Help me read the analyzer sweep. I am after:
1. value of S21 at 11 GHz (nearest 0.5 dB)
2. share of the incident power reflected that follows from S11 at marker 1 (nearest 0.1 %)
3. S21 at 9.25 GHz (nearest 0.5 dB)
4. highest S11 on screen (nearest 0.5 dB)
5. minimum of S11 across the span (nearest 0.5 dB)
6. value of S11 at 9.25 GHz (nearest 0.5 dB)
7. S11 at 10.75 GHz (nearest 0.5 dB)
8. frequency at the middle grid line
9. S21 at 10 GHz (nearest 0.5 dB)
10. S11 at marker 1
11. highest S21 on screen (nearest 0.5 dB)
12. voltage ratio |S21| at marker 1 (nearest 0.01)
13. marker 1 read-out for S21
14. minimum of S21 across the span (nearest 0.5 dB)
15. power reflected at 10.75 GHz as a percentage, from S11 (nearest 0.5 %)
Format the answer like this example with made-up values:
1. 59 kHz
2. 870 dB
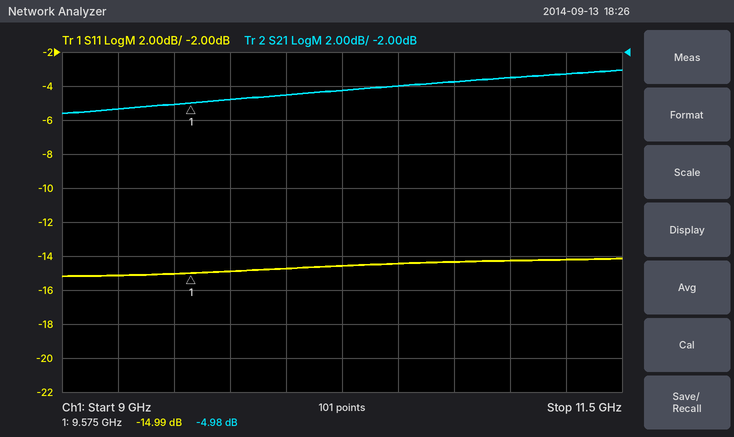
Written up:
1. -3.5 dB
2. 3.2 %
3. -5.5 dB
4. -14.0 dB
5. -15.0 dB
6. -15.0 dB
7. -14.5 dB
8. 10.25 GHz
9. -4.5 dB
10. -14.99 dB
11. -3.0 dB
12. 0.56
13. -4.98 dB
14. -5.5 dB
15. 3.5 %
